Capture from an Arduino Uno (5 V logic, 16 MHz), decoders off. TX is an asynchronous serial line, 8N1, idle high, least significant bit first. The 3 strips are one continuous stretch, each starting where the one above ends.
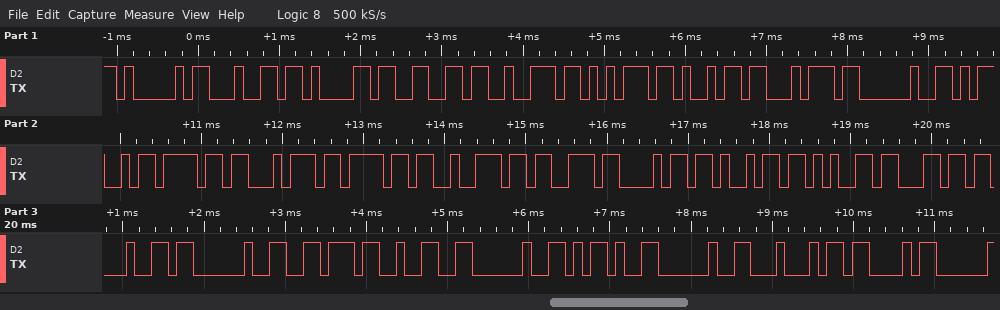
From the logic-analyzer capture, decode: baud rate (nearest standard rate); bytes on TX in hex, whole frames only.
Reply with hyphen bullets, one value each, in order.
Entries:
- 9600 baud
- 41 64 61 66 72 75 69 74 20 4D 6F 74 6F 72 73 68 69 65 6C 64 20 76 32 20 2D 20 44 43
